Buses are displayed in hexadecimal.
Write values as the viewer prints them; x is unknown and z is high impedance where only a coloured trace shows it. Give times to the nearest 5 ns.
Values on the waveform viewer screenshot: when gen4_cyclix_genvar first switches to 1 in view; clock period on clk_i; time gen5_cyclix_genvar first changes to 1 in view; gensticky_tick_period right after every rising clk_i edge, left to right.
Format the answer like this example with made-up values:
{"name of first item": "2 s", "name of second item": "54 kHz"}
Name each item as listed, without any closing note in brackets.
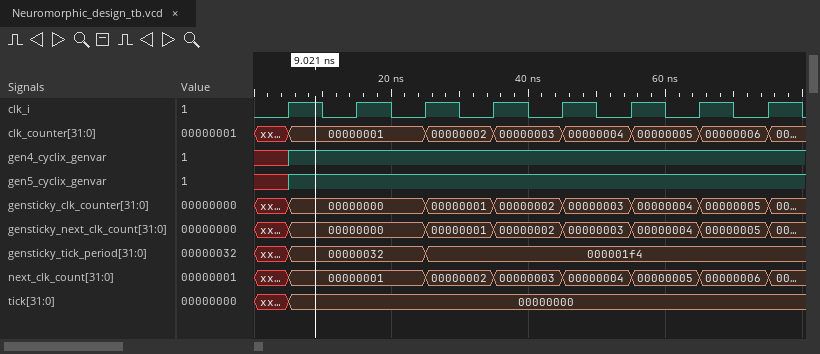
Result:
{"when gen4_cyclix_genvar first switches to 1 in view": "5 ns", "clock period on clk_i": "10 ns", "time gen5_cyclix_genvar first changes to 1 in view": "5 ns", "gensticky_tick_period right after every rising clk_i edge, left to right": "00000032, 00000032, 000001f4, 000001f4, 000001f4, 000001f4, 000001f4, 000001f4"}
